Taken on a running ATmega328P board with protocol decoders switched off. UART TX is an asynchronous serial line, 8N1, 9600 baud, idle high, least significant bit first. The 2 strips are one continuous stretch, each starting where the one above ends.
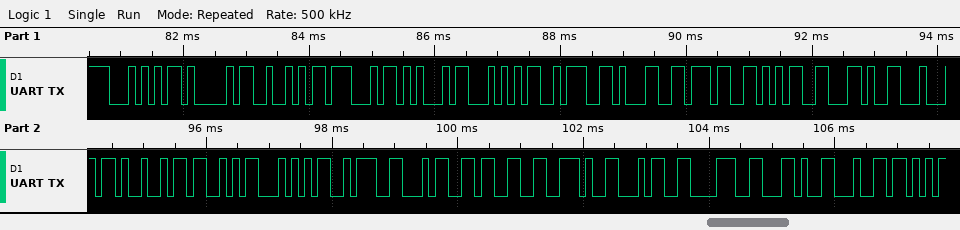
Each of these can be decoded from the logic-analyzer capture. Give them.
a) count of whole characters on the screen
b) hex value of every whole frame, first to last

23
54 41 52 47 45 54 3A 31 37 35 2C 44 49 53 54 3A 34 33 2E 34 38 2C 64
